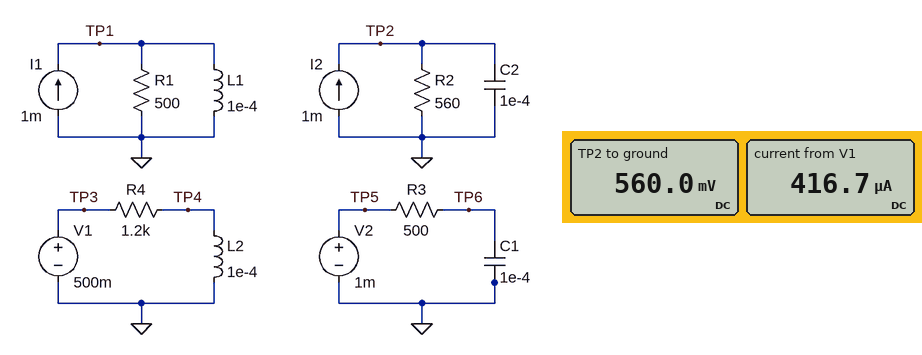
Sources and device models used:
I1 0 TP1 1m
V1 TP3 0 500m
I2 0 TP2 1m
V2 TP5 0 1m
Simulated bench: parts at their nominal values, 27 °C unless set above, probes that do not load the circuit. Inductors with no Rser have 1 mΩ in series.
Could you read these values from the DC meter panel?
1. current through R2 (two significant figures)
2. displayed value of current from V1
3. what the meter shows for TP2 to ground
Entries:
1.0 mA
416.7 µA
560.0 mV
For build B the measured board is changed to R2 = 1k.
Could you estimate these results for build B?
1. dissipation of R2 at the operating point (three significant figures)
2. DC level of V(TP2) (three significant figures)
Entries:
1.00 mW
1.00 V
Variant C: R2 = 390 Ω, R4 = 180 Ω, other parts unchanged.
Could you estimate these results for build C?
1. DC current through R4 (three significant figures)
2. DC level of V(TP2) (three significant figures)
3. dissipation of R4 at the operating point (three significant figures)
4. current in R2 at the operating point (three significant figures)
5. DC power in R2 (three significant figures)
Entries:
2.78 mA
390 mV
1.39 mW
1.00 mA
390 µW
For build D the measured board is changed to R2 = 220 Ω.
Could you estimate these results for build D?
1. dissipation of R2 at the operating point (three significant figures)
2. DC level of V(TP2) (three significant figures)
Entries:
220 µW
220 mV
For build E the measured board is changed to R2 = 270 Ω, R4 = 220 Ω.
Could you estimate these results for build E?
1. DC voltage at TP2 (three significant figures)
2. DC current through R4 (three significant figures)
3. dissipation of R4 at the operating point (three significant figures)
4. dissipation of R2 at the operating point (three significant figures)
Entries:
270 mV
2.27 mA
1.14 mW
270 µW
